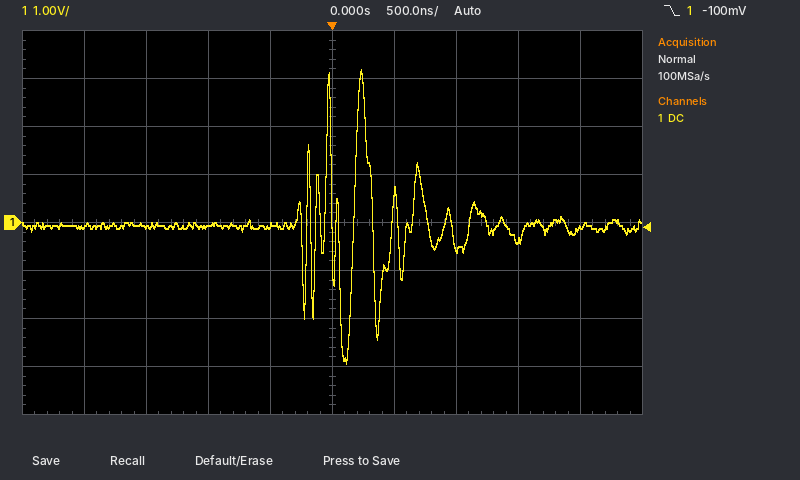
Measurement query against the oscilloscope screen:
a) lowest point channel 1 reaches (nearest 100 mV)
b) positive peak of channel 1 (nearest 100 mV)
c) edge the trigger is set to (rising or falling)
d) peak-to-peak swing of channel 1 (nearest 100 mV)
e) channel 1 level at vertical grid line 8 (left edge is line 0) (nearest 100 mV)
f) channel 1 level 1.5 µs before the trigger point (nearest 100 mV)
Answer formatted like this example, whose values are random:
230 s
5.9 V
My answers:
-2.9 V
3.2 V
falling
6.1 V
-400 mV
-100 mV
